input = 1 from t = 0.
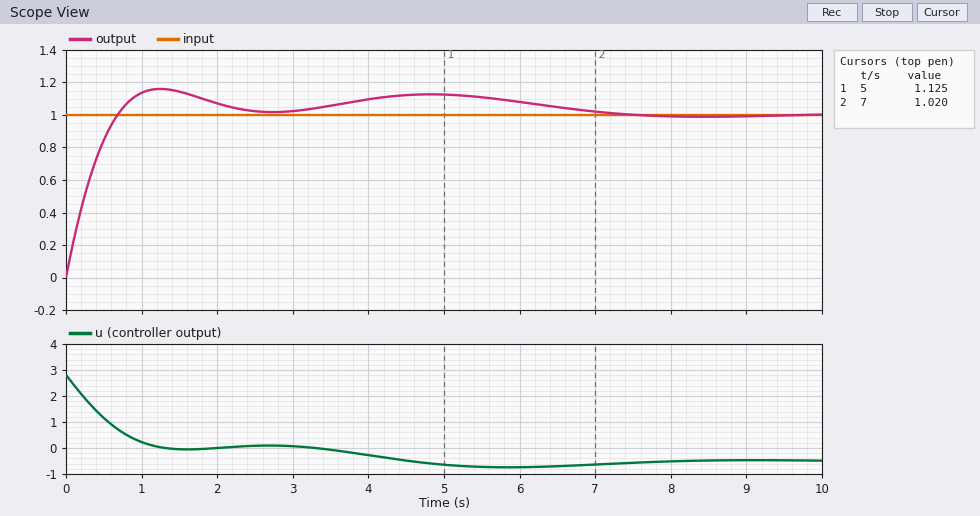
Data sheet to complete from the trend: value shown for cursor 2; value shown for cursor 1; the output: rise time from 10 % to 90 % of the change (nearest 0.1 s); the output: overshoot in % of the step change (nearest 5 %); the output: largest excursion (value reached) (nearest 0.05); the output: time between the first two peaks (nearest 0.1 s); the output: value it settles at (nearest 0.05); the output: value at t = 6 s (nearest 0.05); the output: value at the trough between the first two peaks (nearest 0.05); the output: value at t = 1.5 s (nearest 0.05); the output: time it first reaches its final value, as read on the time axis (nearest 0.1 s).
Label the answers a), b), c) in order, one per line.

a) 1.020
b) 1.125
c) 0.5 s
d) 15 %
e) 1.15
f) 3.6 s
g) 1.00
h) 1.10
i) 1.00
j) 1.15
k) 0.7 s
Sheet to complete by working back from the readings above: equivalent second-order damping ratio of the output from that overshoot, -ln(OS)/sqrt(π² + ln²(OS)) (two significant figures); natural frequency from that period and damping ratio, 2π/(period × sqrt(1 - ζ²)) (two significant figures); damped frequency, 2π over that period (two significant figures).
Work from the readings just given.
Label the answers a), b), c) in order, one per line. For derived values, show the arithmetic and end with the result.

a) ln(0.15) = -1.897; 1.897 / sqrt(9.870 + 3.599) = 0.52
b) 2π / (3.6 × sqrt(1 - 0.52²)) = 2.0 rad/s
c) 2π / 3.6 = 1.7 rad/s
